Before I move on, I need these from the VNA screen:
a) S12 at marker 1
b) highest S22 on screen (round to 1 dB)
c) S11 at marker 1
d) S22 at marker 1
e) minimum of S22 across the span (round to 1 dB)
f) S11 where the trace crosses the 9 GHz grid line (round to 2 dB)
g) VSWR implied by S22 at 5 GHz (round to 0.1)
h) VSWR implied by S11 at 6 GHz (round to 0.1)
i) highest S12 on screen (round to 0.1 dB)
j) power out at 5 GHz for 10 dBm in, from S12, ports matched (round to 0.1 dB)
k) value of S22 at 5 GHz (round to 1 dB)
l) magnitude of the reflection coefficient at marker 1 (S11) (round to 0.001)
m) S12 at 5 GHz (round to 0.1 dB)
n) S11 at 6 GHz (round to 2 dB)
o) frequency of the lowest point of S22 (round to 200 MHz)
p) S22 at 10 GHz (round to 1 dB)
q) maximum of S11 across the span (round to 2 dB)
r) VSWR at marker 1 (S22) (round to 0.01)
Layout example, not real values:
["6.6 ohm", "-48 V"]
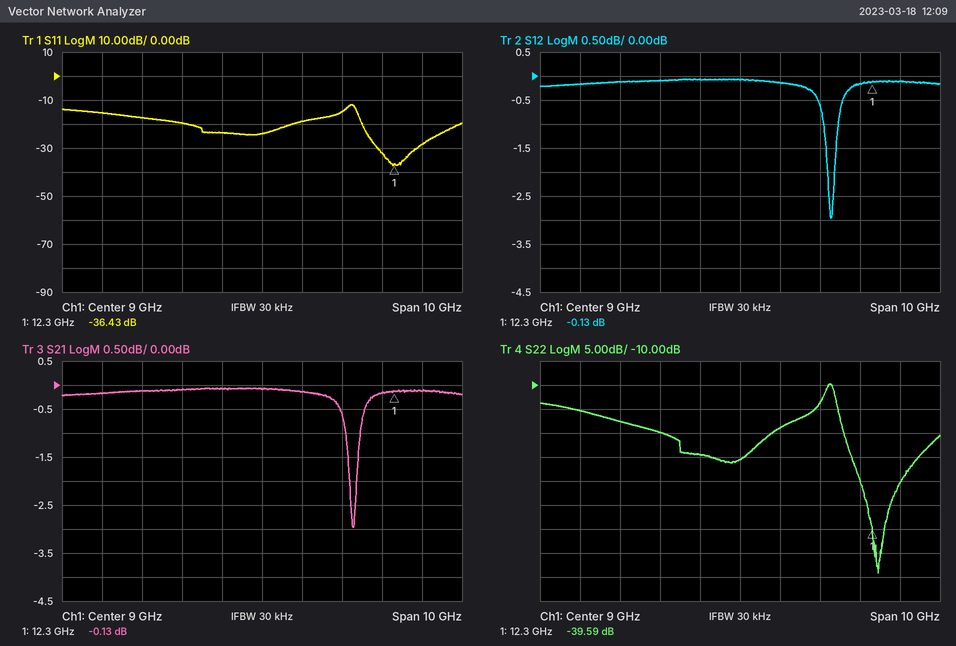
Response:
["-0.13 dB", "-10 dB", "-36.43 dB", "-39.59 dB", "-49 dB", "-24 dB", "1.4", "1.3", "-0.1 dB", "9.8 dBm", "-15 dB", "0.015", "-0.2 dB", "-18 dB", "12.4 GHz", "-19 dB", "-12 dB", "1.02"]
